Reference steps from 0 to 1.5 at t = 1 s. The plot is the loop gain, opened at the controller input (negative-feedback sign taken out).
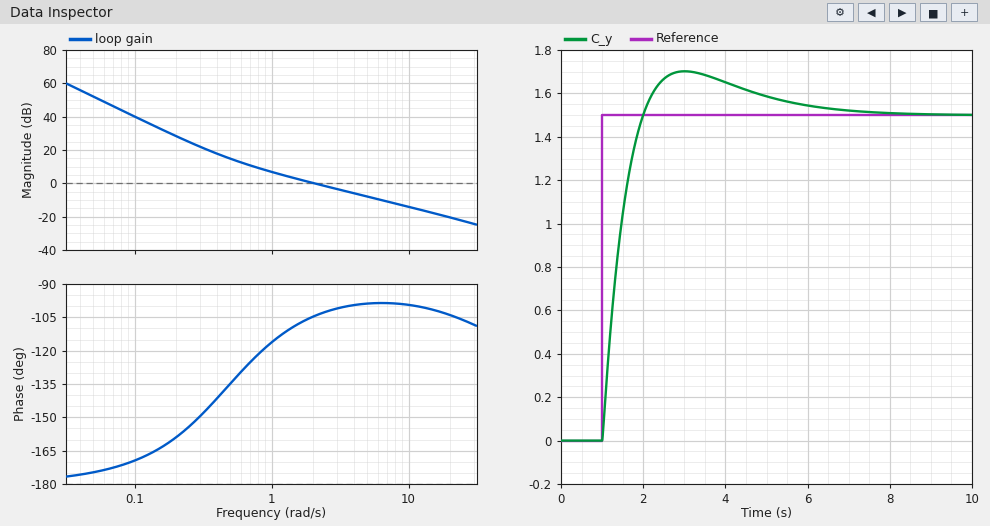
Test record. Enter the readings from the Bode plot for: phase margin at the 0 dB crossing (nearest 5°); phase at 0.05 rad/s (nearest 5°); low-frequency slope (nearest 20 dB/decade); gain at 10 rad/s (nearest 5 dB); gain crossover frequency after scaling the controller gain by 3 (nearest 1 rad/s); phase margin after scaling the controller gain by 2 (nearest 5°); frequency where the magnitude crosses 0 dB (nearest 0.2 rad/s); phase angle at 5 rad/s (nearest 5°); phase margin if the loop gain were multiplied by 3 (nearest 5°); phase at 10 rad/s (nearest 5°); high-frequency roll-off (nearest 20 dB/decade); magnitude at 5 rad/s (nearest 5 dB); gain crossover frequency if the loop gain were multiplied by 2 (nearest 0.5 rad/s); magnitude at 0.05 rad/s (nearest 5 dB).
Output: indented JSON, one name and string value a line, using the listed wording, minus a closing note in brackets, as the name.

{
  "phase margin at the 0 dB crossing": "75°",
  "phase at 0.05 rad/s": "-175°",
  "low-frequency slope": "-40 dB/decade",
  "gain at 10 rad/s": "-15 dB",
  "gain crossover frequency after scaling the controller gain by 3": "6 rad/s",
  "phase margin after scaling the controller gain by 2": "80°",
  "frequency where the magnitude crosses 0 dB": "2.0 rad/s",
  "phase angle at 5 rad/s": "-100°",
  "phase margin if the loop gain were multiplied by 3": "80°",
  "phase at 10 rad/s": "-100°",
  "high-frequency roll-off": "-20 dB/decade",
  "magnitude at 5 rad/s": "-10 dB",
  "gain crossover frequency if the loop gain were multiplied by 2": "4.0 rad/s",
  "magnitude at 0.05 rad/s": "50 dB"
}
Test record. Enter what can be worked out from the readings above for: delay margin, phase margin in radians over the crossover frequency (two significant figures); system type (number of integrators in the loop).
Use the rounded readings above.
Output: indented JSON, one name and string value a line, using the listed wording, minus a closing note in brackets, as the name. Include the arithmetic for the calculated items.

{
  "delay margin, phase margin in radians over the crossover frequency": "75 × π / 180 / 2 = 0.65 s",
  "system type": "2"
}
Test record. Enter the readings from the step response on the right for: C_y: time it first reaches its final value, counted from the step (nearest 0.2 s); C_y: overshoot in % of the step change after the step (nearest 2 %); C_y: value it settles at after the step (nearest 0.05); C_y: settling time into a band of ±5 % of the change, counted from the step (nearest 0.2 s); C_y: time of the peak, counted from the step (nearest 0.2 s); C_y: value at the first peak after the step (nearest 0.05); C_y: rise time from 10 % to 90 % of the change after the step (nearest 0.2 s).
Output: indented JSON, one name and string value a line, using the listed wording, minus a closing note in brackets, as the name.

{
  "C_y: time it first reaches its final value, counted from the step": "1.0 s",
  "C_y: overshoot in % of the step change after the step": "14 %",
  "C_y: value it settles at after the step": "1.50",
  "C_y: settling time into a band of ±5 % of the change, counted from the step": "4.2 s",
  "C_y: time of the peak, counted from the step": "2.0 s",
  "C_y: value at the first peak after the step": "1.70",
  "C_y: rise time from 10 % to 90 % of the change after the step": "0.8 s"
}
